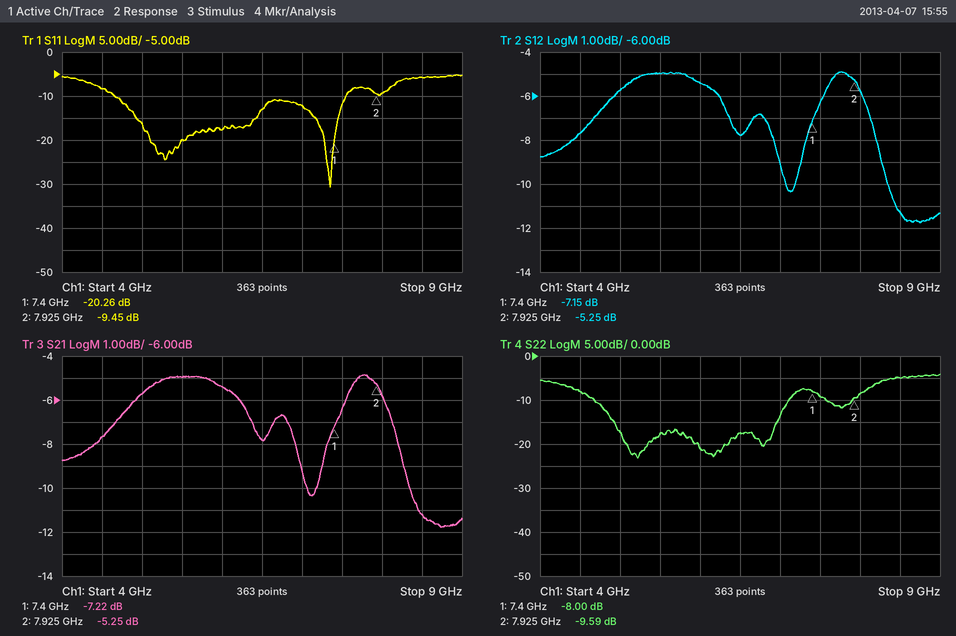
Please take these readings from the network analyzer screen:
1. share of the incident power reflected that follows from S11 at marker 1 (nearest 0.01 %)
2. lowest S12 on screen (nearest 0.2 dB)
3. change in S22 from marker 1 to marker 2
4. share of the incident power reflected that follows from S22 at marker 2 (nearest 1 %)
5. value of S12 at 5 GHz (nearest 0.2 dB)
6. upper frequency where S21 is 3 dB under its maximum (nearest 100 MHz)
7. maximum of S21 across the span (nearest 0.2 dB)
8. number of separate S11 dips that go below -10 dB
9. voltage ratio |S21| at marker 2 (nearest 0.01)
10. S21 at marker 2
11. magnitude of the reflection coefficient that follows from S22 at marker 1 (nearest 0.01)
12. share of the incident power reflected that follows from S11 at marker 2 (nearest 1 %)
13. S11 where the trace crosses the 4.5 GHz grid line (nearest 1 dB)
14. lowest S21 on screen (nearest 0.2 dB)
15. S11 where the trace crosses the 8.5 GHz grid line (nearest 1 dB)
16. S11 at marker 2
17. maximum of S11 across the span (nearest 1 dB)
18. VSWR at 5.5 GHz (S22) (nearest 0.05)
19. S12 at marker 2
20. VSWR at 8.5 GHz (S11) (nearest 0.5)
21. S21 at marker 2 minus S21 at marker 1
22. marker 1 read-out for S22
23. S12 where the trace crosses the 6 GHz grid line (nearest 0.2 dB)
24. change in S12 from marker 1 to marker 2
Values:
0.94 %
-11.8 dB
-1.59 dB
11 %
-5.8 dB
8.2 GHz
-4.8 dB
2
0.55
-5.25 dB
0.40
11 %
-8 dB
-11.8 dB
-6 dB
-9.45 dB
-5 dB
1.30
-5.25 dB
3.0
1.97 dB
-8.00 dB
-5.4 dB
1.90 dB
